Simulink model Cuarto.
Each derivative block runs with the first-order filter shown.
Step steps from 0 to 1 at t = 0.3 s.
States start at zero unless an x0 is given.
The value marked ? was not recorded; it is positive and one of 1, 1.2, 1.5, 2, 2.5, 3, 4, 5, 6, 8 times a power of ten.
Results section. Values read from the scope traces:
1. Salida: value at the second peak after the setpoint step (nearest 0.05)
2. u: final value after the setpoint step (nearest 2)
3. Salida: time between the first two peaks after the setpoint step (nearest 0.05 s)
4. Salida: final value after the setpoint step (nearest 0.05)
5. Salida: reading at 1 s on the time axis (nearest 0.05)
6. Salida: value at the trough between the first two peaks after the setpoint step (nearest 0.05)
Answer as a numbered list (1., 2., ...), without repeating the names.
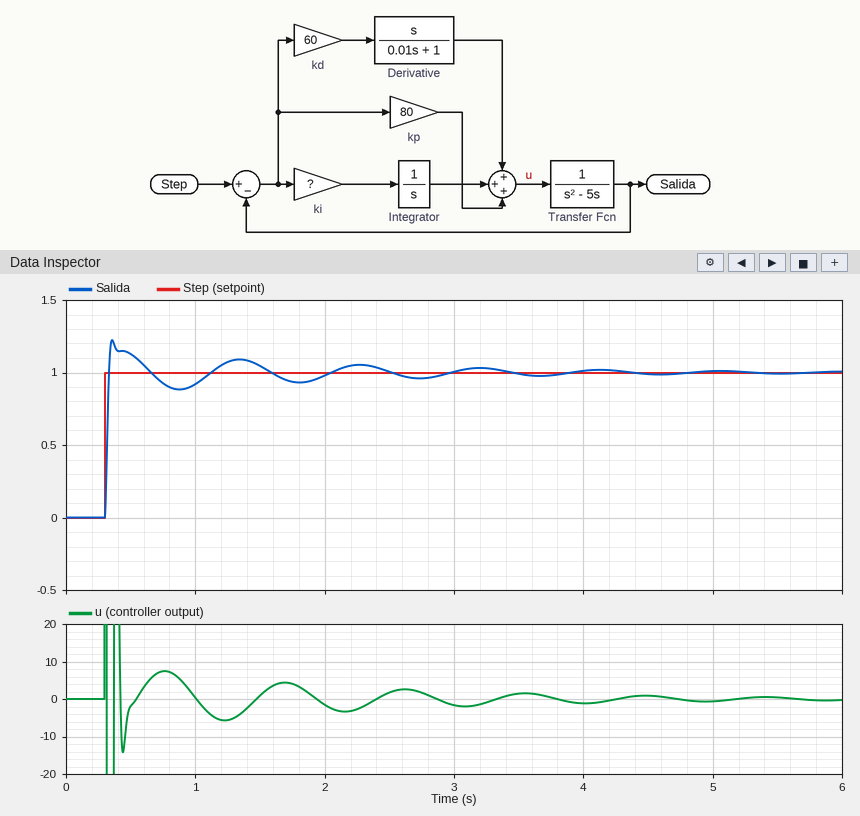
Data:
1. 1.10
2. 0
3. 1.00 s
4. 1.00
5. 0.90
6. 0.90
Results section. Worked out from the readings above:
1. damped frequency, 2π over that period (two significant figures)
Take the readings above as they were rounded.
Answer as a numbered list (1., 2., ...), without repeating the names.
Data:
1. 6.3 rad/s
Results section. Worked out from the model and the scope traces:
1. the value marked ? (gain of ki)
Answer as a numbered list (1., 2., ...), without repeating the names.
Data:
1. 2500
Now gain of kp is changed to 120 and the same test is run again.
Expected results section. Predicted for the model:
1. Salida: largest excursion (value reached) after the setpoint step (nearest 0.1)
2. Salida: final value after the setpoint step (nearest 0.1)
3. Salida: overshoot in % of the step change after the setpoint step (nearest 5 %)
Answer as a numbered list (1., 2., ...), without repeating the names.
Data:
1. 1.2
2. 1.0
3. 25 %
